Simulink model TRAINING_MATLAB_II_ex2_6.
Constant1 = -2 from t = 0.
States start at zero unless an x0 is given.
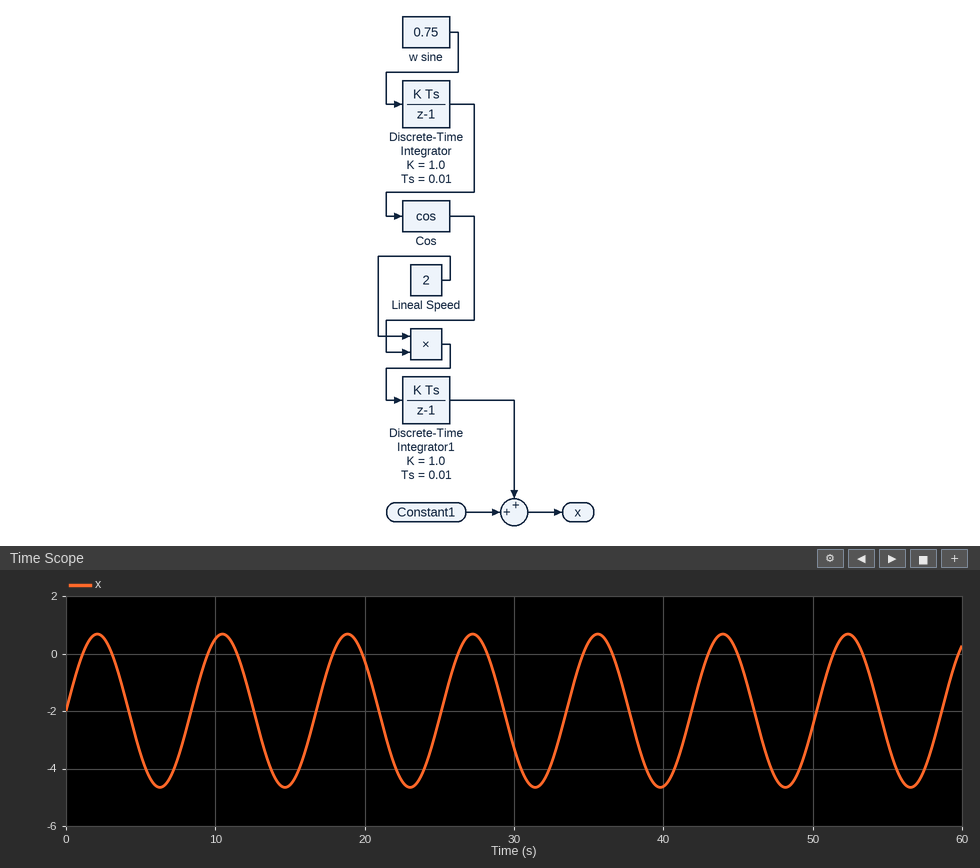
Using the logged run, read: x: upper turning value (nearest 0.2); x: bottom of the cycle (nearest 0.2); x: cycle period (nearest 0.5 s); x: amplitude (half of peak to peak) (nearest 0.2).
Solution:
0.6
-4.6
8.5 s
2.6
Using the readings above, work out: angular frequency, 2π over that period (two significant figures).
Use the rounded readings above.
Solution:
0.74 rad/s
